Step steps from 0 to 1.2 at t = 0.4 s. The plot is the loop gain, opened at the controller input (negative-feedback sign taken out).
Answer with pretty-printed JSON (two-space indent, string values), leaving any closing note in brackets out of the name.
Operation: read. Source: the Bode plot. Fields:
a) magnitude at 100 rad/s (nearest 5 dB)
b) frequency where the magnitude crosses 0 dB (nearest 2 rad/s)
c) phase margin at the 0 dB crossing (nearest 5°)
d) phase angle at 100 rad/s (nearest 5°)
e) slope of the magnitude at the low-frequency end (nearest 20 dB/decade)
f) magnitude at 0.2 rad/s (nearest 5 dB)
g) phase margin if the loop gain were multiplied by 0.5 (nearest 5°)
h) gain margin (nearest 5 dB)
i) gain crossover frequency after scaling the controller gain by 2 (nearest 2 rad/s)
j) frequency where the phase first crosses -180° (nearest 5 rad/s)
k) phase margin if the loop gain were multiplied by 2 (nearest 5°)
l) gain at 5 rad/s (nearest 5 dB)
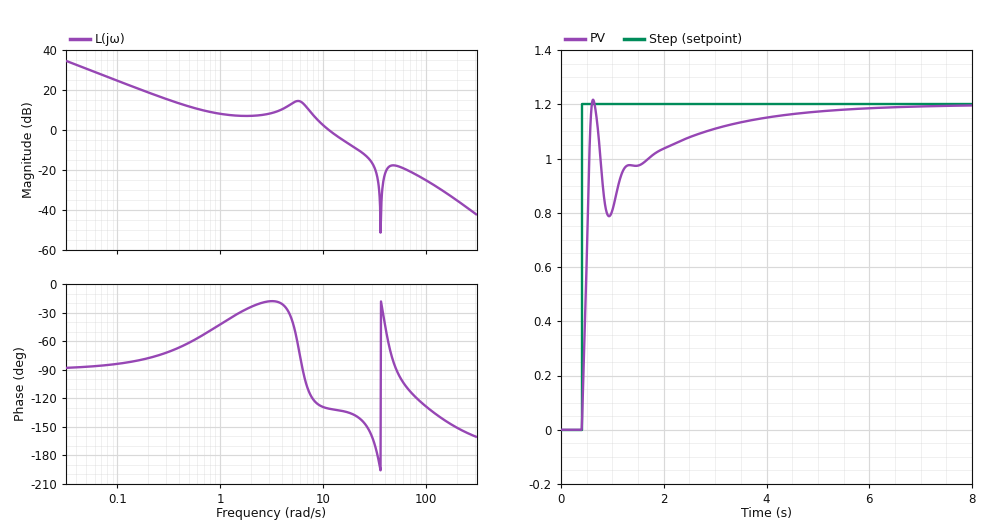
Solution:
{
  "magnitude at 100 rad/s": "-25 dB",
  "frequency where the magnitude crosses 0 dB": "12 rad/s",
  "phase margin at the 0 dB crossing": "50°",
  "phase angle at 100 rad/s": "-130°",
  "slope of the magnitude at the low-frequency end": "-20 dB/decade",
  "magnitude at 0.2 rad/s": "20 dB",
  "phase margin if the loop gain were multiplied by 0.5": "55°",
  "gain margin": "25 dB",
  "gain crossover frequency after scaling the controller gain by 2": "16 rad/s",
  "frequency where the phase first crosses -180°": "35 rad/s",
  "phase margin if the loop gain were multiplied by 2": "45°",
  "gain at 5 rad/s": "15 dB"
}
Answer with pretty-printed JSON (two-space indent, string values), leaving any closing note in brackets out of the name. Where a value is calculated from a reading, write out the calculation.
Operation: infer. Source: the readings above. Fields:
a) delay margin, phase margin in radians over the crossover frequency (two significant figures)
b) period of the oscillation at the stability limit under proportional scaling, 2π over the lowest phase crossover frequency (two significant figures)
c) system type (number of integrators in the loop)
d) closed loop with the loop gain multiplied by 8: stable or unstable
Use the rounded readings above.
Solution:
{
  "delay margin, phase margin in radians over the crossover frequency": "50 × π / 180 / 12 = 0.073 s",
  "period of the oscillation at the stability limit under proportional scaling, 2π over the lowest phase crossover frequency": "2π / 35 = 0.18 s",
  "system type": "1",
  "closed loop with the loop gain multiplied by 8: stable or unstable": "stable"
}
